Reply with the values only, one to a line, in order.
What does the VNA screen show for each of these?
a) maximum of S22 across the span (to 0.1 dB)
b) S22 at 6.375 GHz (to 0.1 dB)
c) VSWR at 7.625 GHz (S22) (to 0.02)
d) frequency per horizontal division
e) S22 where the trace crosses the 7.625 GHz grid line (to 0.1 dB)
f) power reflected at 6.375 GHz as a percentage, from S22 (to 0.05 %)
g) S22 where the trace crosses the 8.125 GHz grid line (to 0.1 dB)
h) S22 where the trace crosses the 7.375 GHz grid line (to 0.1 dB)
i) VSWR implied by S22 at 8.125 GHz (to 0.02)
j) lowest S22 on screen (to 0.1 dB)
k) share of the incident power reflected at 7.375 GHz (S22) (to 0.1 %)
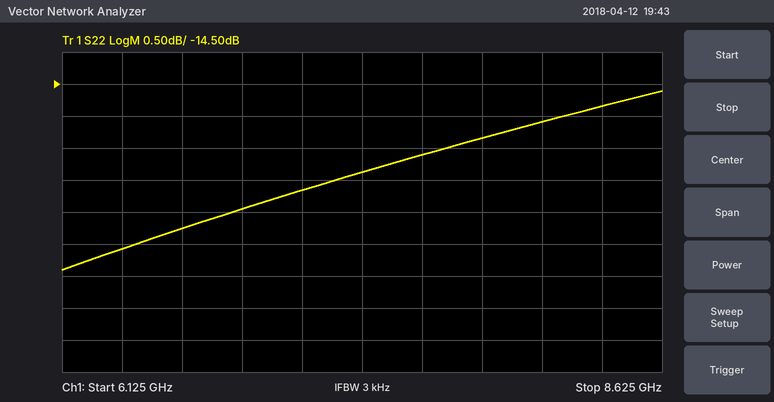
-14.6 dB
-17.1 dB
1.40
250 MHz
-15.6 dB
1.95 %
-15.1 dB
-15.9 dB
1.42
-17.4 dB
2.6 %
